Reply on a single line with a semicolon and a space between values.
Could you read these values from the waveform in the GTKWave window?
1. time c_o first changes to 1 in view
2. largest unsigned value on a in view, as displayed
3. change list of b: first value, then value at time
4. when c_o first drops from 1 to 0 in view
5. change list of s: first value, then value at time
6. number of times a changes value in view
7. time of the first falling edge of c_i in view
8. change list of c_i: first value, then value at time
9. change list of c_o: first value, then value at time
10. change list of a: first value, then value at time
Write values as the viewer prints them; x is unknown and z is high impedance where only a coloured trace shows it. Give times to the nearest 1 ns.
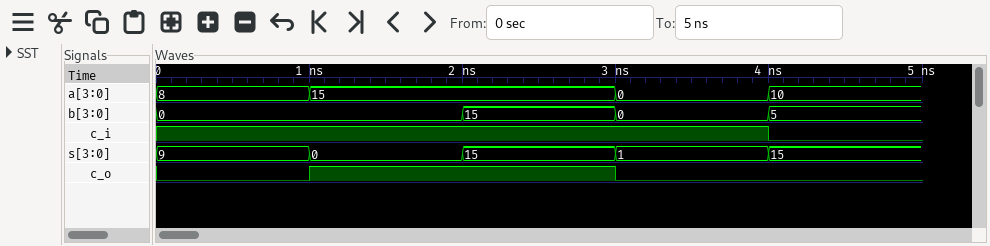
1 ns; 15; 0, 15 at 2 ns, 0 at 3 ns, 5 at 4 ns; 3 ns; 9, 0 at 1 ns, 15 at 2 ns, 1 at 3 ns, 15 at 4 ns; 3; 4 ns; 1, 0 at 4 ns; 0, 1 at 1 ns, 0 at 3 ns; 8, 15 at 1 ns, 0 at 3 ns, 10 at 4 ns
